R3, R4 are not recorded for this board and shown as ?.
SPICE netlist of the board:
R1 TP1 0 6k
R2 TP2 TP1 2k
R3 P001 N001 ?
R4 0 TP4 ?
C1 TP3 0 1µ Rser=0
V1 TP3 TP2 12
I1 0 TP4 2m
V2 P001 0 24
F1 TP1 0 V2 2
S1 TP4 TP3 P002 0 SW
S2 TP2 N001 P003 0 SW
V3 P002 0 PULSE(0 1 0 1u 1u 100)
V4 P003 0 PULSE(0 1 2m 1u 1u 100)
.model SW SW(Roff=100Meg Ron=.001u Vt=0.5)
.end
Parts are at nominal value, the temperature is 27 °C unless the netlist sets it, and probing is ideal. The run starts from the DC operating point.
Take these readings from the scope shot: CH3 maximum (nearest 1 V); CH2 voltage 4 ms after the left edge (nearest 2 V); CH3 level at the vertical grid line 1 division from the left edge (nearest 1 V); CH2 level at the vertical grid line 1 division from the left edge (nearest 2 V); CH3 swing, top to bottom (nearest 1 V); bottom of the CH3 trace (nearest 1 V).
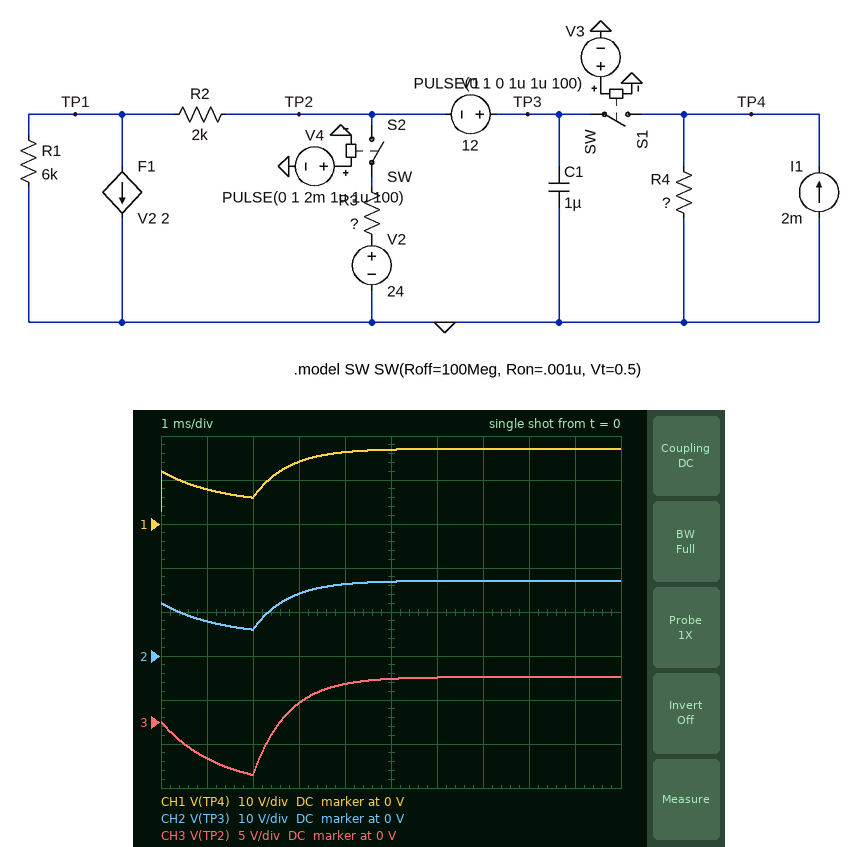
5 V
16 V
-4 V
8 V
11 V
-6 V
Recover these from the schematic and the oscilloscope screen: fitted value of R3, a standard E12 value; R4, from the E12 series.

4.7 kΩ
1.5 kΩ
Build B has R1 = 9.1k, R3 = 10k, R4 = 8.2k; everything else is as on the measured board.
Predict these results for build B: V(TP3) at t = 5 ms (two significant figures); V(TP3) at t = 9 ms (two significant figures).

23 V
26 V
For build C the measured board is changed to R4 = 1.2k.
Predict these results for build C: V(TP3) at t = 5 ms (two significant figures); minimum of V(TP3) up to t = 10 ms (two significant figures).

15 V
4.9 V
